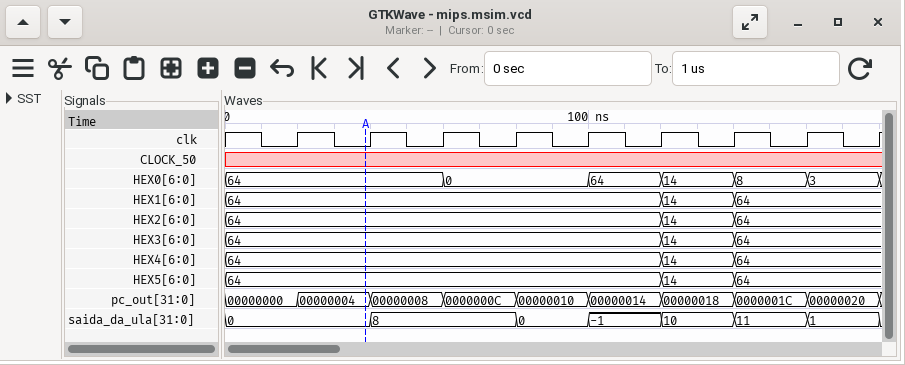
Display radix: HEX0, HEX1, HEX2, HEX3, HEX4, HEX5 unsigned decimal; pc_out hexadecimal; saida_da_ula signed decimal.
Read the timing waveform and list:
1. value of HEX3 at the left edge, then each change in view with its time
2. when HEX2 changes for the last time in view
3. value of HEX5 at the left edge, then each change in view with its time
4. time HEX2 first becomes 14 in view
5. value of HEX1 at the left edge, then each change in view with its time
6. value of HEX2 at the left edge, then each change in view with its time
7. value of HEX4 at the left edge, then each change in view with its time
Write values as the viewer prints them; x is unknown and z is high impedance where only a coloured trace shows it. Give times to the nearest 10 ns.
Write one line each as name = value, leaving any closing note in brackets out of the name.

value of HEX3 at the left edge, then each change in view with its time = 64, 14 at 120 ns, 64 at 140 ns
when HEX2 changes for the last time in view = 140 ns
value of HEX5 at the left edge, then each change in view with its time = 64, 14 at 120 ns, 64 at 140 ns
time HEX2 first becomes 14 in view = 120 ns
value of HEX1 at the left edge, then each change in view with its time = 64, 14 at 120 ns, 64 at 140 ns
value of HEX2 at the left edge, then each change in view with its time = 64, 14 at 120 ns, 64 at 140 ns
value of HEX4 at the left edge, then each change in view with its time = 64, 14 at 120 ns, 64 at 140 ns
